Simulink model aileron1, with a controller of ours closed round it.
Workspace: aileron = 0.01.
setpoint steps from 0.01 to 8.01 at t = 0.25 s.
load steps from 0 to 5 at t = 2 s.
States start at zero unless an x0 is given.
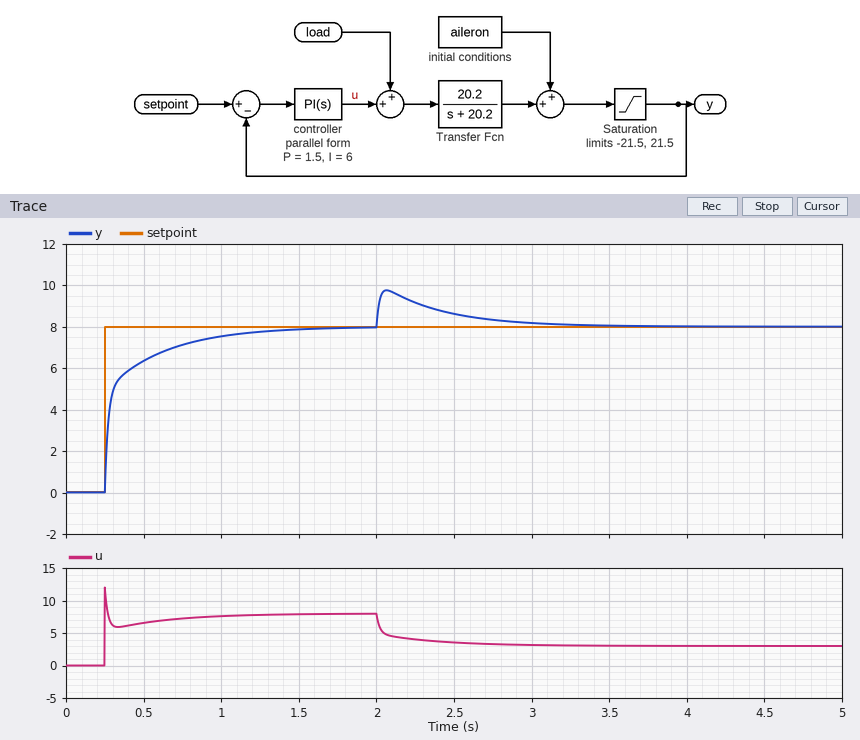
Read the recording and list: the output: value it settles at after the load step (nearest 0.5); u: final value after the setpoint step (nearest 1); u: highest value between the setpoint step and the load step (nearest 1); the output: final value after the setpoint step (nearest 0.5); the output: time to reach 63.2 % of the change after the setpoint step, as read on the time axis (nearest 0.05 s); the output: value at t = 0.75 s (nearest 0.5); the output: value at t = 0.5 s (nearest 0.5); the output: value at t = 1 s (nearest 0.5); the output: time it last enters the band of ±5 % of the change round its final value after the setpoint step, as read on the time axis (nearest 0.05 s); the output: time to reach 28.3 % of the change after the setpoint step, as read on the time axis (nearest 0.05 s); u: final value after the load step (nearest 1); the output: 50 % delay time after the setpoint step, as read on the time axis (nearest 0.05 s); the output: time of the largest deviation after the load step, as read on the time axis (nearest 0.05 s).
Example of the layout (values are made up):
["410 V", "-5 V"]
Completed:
["8.0", "8", "12", "8.0", "0.30 s", "7.0", "6.5", "7.5", "1.05 s", "0.25 s", "3", "0.30 s", "2.05 s"]
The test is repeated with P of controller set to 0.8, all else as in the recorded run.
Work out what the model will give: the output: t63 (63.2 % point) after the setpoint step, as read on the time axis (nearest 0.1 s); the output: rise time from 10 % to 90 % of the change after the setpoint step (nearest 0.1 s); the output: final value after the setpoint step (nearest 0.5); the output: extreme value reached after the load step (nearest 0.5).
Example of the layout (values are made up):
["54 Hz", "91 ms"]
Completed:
["0.4 s", "0.5 s", "8.0", "10.5"]
